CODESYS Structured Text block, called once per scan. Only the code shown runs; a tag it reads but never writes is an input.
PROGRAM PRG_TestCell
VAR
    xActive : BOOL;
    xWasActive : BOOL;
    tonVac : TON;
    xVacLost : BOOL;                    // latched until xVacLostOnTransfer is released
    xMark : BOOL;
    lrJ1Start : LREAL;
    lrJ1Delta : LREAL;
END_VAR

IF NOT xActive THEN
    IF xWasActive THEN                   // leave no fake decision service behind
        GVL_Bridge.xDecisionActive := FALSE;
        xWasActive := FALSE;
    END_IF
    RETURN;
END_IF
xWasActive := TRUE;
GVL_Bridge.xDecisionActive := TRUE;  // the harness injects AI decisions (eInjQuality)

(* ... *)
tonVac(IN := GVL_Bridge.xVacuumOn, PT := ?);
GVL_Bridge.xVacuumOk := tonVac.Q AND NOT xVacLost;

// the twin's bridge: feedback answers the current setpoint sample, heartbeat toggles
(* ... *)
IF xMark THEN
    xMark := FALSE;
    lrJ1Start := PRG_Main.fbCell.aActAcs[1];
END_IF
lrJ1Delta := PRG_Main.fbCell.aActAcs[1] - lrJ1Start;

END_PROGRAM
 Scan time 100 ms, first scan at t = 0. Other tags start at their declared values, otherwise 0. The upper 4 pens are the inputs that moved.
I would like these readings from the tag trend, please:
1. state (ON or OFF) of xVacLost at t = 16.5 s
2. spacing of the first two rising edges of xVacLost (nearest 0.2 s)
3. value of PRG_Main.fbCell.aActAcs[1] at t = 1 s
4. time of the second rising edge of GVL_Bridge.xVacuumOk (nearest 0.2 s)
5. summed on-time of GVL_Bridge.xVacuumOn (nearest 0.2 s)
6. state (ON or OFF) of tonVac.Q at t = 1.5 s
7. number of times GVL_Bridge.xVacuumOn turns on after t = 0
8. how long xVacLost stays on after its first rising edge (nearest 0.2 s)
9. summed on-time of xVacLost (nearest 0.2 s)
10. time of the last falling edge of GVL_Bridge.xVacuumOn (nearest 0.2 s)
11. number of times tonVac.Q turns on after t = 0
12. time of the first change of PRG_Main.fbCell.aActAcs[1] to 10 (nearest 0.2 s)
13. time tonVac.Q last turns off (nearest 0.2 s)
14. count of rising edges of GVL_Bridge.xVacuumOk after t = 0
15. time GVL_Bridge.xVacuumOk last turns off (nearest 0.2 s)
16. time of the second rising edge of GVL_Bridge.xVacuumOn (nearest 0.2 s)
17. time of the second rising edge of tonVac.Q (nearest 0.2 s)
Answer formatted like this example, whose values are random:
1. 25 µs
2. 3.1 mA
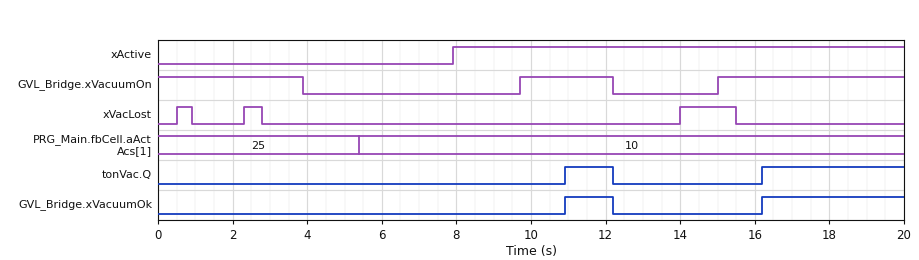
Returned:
1. OFF
2. 1.8 s
3. 25
4. 16.2 s
5. 11.4 s
6. OFF
7. 2
8. 0.4 s
9. 2.4 s
10. 12.2 s
11. 2
12. 5.4 s
13. 12.2 s
14. 2
15. 12.2 s
16. 15.0 s
17. 16.2 s
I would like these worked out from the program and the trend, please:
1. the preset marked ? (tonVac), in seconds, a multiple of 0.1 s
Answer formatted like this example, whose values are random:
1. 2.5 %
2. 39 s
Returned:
1. 1.2 s
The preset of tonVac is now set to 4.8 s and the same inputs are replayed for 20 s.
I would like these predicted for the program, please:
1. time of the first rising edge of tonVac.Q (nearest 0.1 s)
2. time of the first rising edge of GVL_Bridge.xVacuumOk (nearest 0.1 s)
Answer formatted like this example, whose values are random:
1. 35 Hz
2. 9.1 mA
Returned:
1. 19.8 s
2. 19.8 s
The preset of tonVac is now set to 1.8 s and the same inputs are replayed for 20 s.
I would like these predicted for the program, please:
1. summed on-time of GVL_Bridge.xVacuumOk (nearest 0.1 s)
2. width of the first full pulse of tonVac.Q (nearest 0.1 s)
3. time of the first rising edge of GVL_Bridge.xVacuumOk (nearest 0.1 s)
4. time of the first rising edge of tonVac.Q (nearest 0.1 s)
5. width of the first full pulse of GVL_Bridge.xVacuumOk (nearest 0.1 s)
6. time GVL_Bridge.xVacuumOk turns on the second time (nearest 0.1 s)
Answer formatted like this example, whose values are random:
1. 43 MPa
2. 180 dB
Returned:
1. 3.9 s
2. 0.7 s
3. 11.5 s
4. 11.5 s
5. 0.7 s
6. 16.8 s
